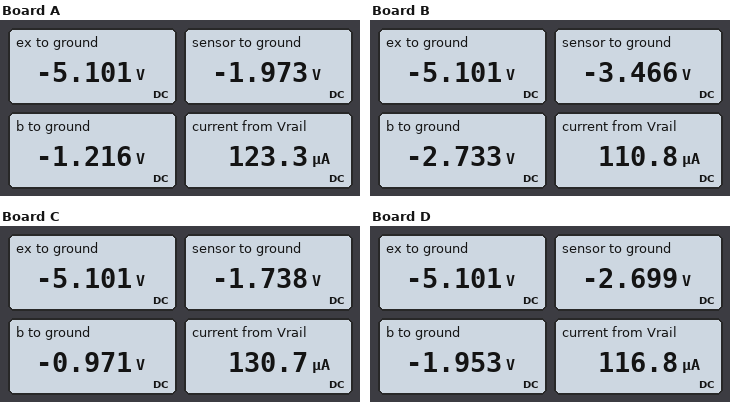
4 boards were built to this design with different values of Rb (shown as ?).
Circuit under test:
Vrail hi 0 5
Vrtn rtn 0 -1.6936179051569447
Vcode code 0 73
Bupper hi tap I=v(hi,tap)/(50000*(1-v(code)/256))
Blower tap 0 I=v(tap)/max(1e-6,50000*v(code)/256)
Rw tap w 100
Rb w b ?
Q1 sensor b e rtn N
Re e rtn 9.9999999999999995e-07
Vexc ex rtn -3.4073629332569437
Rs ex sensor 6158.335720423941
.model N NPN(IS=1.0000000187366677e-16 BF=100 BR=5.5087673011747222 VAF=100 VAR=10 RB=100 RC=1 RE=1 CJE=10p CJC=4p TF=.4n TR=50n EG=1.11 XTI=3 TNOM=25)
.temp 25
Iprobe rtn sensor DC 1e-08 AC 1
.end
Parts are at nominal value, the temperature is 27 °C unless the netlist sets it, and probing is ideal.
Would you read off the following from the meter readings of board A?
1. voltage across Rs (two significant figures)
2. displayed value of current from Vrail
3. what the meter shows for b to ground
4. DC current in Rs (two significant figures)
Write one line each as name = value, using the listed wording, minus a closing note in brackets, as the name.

voltage across Rs = 3.1 V
displayed value of current from Vrail = 123.3 µA
what the meter shows for b to ground = -1.216 V
DC current in Rs = 510 µA
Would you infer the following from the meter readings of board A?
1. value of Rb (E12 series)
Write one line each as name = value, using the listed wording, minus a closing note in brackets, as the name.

value of Rb = 22 kΩ
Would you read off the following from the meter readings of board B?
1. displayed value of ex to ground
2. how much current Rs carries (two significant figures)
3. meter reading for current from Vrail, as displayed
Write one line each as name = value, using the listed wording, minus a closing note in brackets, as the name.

displayed value of ex to ground = -5.101 V
how much current Rs carries = 270 µA
meter reading for current from Vrail, as displayed = 110.8 µA
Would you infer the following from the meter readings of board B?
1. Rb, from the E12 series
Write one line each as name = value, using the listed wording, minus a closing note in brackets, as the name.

Rb, from the E12 series = 100 kΩ
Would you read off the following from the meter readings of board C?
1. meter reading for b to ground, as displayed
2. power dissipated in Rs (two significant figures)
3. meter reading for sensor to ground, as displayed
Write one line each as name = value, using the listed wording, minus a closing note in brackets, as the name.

meter reading for b to ground, as displayed = -0.971 V
power dissipated in Rs = 1.8 mW
meter reading for sensor to ground, as displayed = -1.738 V
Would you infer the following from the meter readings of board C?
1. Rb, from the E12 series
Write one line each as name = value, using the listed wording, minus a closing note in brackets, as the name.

Rb, from the E12 series = 12 kΩ
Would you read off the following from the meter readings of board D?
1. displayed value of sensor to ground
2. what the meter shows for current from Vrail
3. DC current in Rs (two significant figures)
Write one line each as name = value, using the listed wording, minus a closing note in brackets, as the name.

displayed value of sensor to ground = -2.699 V
what the meter shows for current from Vrail = 116.8 µA
DC current in Rs = 390 µA
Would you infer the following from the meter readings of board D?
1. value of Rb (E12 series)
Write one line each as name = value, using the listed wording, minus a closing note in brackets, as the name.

value of Rb = 47 kΩ
